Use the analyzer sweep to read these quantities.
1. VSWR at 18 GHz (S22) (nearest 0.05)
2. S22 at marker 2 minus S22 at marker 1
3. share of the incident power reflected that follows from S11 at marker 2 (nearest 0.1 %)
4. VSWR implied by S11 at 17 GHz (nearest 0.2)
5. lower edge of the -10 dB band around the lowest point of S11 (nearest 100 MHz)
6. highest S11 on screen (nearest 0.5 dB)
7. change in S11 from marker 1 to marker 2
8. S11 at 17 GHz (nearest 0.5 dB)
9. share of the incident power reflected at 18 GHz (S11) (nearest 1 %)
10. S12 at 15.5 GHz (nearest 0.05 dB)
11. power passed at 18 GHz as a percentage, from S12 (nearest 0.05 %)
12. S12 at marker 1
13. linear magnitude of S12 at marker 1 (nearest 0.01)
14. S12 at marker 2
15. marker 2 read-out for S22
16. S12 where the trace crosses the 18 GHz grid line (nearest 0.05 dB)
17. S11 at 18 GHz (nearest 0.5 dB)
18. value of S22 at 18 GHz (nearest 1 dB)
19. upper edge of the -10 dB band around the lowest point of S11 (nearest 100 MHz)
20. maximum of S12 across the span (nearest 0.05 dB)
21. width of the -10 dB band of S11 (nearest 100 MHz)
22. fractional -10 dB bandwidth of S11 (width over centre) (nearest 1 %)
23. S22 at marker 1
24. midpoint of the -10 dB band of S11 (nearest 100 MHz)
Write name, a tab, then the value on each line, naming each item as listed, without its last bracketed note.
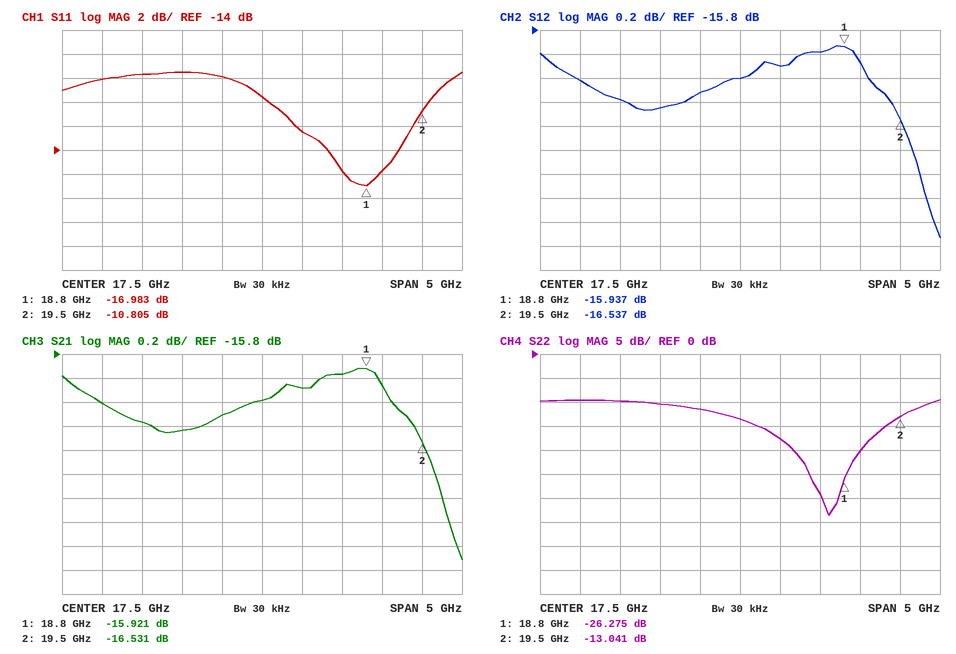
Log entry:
VSWR at 18 GHz (S22)	1.30
S22 at marker 2 minus S22 at marker 1	13.234 dB
share of the incident power reflected that follows from S11 at marker 2	8.3 %
VSWR implied by S11 at 17 GHz	2.4
lower edge of the -10 dB band around the lowest point of S11	17.6 GHz
highest S11 on screen	-7.5 dB
change in S11 from marker 1 to marker 2	6.178 dB
S11 at 17 GHz	-8.0 dB
share of the incident power reflected at 18 GHz (S11)	6 %
S12 at 15.5 GHz	-16.20 dB
power passed at 18 GHz as a percentage, from S12	2.45 %
S12 at marker 1	-15.937 dB
linear magnitude of S12 at marker 1	0.16
S12 at marker 2	-16.537 dB
marker 2 read-out for S22	-13.041 dB
S12 where the trace crosses the 18 GHz grid line	-16.10 dB
S11 at 18 GHz	-12.5 dB
value of S22 at 18 GHz	-18 dB
upper edge of the -10 dB band around the lowest point of S11	19.6 GHz
maximum of S12 across the span	-15.95 dB
width of the -10 dB band of S11	2.0 GHz
fractional -10 dB bandwidth of S11 (width over centre)	11 %
S22 at marker 1	-26.275 dB
midpoint of the -10 dB band of S11	18.6 GHz
